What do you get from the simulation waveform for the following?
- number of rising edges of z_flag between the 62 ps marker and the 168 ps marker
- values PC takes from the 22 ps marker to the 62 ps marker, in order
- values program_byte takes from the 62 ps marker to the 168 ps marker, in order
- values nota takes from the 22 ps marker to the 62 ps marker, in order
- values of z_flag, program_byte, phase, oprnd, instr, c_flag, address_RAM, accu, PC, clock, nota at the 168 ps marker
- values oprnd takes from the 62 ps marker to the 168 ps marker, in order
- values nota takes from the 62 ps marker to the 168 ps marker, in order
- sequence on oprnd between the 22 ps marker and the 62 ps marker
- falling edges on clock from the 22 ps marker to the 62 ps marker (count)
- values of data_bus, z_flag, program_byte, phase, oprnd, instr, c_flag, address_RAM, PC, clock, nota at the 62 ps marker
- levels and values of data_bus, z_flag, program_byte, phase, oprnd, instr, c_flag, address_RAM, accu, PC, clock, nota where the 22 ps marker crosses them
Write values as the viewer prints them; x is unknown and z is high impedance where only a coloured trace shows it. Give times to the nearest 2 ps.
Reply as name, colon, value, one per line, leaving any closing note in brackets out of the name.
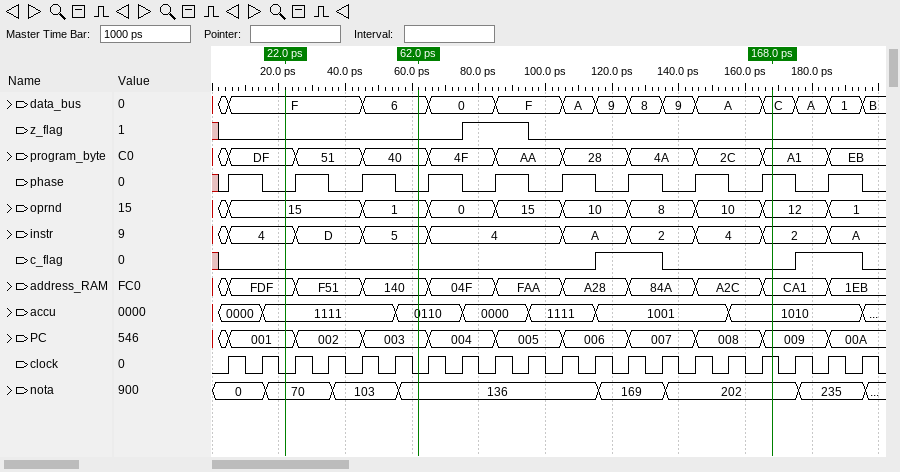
number of rising edges of z_flag between the 62 ps marker and the 168 ps marker: 1
values PC takes from the 22 ps marker to the 62 ps marker, in order: 001, 002, 003
values program_byte takes from the 62 ps marker to the 168 ps marker, in order: 40, 4F, AA, 28, 4A, 2C, A1
values nota takes from the 22 ps marker to the 62 ps marker, in order: 70, 103, 136
values of z_flag, program_byte, phase, oprnd, instr, c_flag, address_RAM, accu, PC, clock, nota at the 168 ps marker: z_flag=0, program_byte=A1, phase=1, oprnd=12, instr=2, c_flag=0, address_RAM=CA1, accu=1010, PC=009, clock=1, nota=202
values oprnd takes from the 62 ps marker to the 168 ps marker, in order: 1, 0, 15, 10, 8, 10, 12
values nota takes from the 62 ps marker to the 168 ps marker, in order: 136, 169, 202
sequence on oprnd between the 22 ps marker and the 62 ps marker: 15, 1
falling edges on clock from the 22 ps marker to the 62 ps marker: 4
values of data_bus, z_flag, program_byte, phase, oprnd, instr, c_flag, address_RAM, PC, clock, nota at the 62 ps marker: data_bus=6, z_flag=0, program_byte=40, phase=0, oprnd=1, instr=5, c_flag=0, address_RAM=140, PC=003, clock=0, nota=136
levels and values of data_bus, z_flag, program_byte, phase, oprnd, instr, c_flag, address_RAM, accu, PC, clock, nota where the 22 ps marker crosses them: data_bus=F, z_flag=0, program_byte=DF, phase=0, oprnd=15, instr=4, c_flag=0, address_RAM=FDF, accu=1111, PC=001, clock=0, nota=70
